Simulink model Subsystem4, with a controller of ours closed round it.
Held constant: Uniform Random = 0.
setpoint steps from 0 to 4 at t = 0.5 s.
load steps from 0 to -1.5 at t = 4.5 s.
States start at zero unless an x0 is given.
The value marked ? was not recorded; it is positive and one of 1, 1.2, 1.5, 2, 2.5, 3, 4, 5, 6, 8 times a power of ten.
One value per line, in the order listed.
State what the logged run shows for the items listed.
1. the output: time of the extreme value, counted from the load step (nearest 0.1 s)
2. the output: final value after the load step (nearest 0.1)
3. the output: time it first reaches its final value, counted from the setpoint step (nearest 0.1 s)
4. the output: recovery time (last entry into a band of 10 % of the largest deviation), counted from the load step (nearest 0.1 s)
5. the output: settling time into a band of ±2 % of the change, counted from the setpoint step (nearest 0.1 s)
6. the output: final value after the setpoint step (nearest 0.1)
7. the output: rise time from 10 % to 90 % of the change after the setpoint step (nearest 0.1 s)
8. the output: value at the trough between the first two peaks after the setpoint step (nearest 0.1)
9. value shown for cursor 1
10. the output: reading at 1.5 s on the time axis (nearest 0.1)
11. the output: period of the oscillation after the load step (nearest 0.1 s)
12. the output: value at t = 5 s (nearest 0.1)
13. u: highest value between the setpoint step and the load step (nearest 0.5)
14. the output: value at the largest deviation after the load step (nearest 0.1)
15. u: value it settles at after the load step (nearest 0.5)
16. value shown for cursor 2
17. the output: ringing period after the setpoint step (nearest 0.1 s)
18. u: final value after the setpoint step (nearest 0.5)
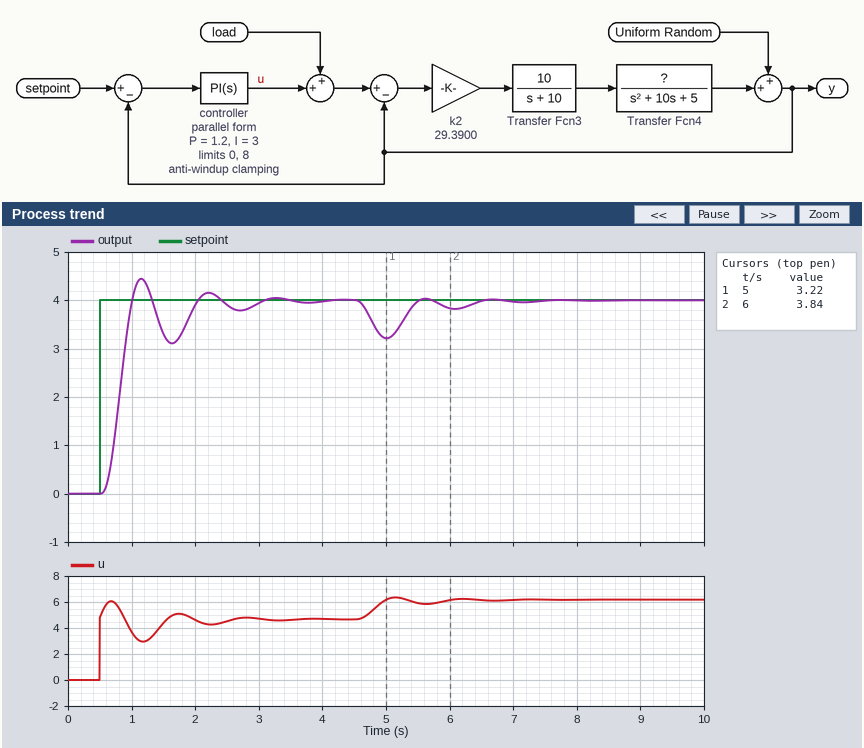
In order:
0.5 s
4.0
0.5 s
1.9 s
2.5 s
4.0
0.3 s
3.1
3.22
3.3
1.1 s
3.2
6.0
3.2
6.0
3.84
1.1 s
4.5
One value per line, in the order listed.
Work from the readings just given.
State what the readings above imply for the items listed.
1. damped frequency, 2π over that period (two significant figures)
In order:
5.7 rad/s
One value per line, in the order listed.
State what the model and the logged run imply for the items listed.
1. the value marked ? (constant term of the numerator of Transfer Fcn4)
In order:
1
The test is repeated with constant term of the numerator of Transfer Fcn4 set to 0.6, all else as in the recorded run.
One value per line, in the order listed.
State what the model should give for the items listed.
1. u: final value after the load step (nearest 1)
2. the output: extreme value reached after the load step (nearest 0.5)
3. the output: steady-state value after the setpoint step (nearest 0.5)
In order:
7
3.5
4.0
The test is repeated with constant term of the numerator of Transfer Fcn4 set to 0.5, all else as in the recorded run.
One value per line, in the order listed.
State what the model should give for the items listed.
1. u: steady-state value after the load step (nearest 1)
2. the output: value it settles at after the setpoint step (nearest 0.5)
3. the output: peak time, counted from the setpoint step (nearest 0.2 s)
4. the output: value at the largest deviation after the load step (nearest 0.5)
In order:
7
4.0
1.0 s
3.5
